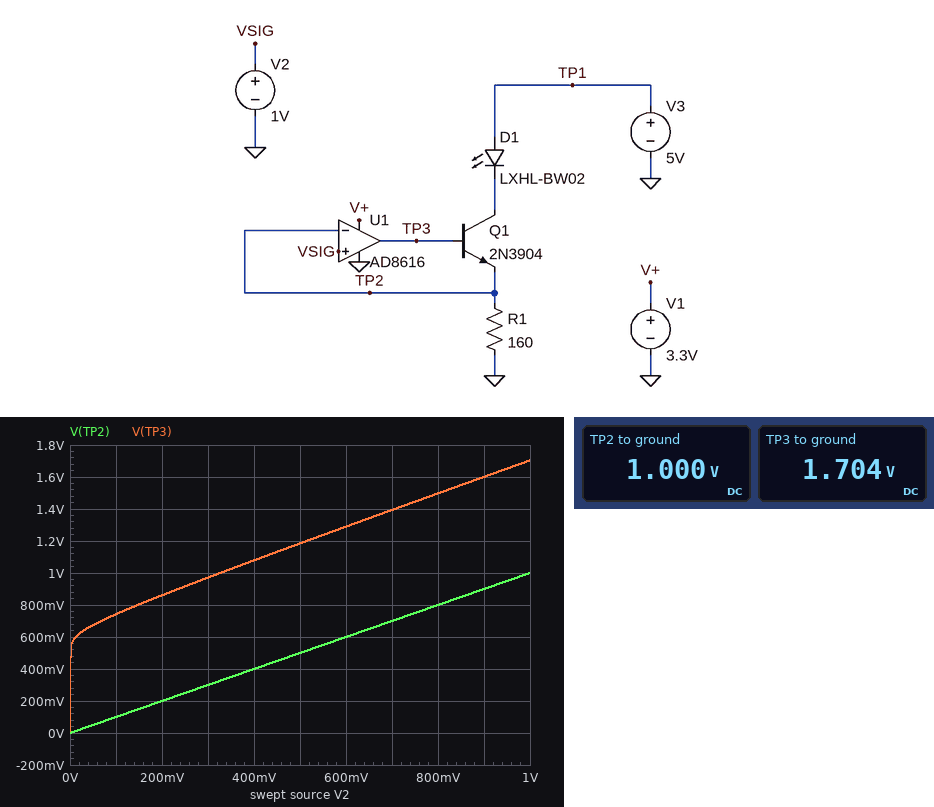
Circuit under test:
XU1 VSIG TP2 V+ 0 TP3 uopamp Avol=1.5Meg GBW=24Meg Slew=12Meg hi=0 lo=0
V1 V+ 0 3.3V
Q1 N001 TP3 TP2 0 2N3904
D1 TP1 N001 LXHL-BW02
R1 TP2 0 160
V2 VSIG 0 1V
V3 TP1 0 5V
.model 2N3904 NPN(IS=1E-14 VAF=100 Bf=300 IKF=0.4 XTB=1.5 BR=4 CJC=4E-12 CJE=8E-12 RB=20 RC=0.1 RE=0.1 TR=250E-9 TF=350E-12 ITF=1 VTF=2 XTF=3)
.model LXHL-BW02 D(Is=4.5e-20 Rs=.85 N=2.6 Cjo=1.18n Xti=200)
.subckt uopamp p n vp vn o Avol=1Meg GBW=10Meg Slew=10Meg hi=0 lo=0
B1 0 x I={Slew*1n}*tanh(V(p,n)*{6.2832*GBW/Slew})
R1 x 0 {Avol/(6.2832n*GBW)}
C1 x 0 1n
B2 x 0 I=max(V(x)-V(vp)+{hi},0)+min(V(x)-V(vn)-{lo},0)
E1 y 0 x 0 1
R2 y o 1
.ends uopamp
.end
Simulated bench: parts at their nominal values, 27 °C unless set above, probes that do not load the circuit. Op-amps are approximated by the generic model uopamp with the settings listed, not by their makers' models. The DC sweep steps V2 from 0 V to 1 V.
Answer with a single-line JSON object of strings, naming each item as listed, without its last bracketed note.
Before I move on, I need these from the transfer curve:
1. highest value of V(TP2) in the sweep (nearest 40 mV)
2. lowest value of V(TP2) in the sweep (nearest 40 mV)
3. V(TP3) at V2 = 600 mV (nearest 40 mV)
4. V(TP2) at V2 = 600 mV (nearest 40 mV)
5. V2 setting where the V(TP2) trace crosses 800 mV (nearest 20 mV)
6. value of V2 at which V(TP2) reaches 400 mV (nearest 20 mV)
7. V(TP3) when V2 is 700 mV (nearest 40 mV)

{"highest value of V(TP2) in the sweep": "1.00 V", "lowest value of V(TP2) in the sweep": "0 V", "V(TP3) at V2 = 600 mV": "1.28 V", "V(TP2) at V2 = 600 mV": "600 mV", "V2 setting where the V(TP2) trace crosses 800 mV": "800 mV", "value of V2 at which V(TP2) reaches 400 mV": "400 mV", "V(TP3) when V2 is 700 mV": "1.40 V"}
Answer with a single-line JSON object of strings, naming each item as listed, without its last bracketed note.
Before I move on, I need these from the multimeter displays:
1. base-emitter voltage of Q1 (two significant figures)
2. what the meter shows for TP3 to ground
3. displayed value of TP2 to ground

{"base-emitter voltage of Q1": "700 mV", "what the meter shows for TP3 to ground": "1.704 V", "displayed value of TP2 to ground": "1.000 V"}
